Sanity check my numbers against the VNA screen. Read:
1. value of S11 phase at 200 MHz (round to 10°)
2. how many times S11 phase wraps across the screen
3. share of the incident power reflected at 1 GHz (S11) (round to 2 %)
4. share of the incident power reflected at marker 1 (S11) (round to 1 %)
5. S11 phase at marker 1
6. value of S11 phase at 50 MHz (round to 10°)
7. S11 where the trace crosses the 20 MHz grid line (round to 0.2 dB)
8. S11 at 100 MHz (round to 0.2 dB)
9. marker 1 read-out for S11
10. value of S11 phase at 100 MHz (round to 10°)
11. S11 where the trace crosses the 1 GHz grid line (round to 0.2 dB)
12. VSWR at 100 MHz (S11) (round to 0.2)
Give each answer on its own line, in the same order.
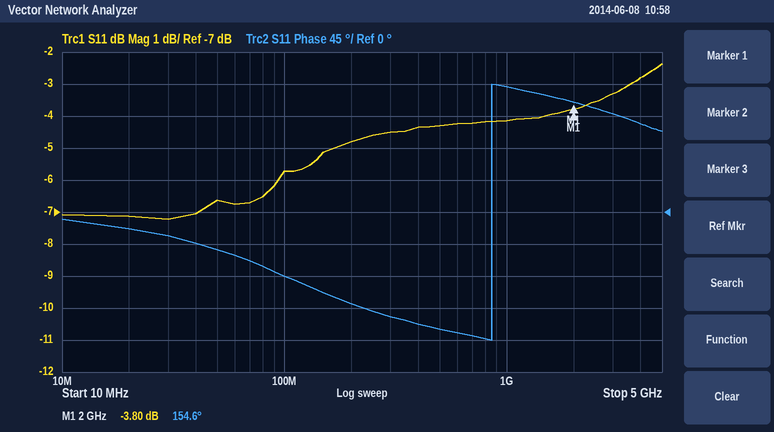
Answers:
-130°
1
38 %
42 %
154.6°
-50°
-7.2 dB
-5.8 dB
-3.80 dB
-90°
-4.2 dB
3.2
